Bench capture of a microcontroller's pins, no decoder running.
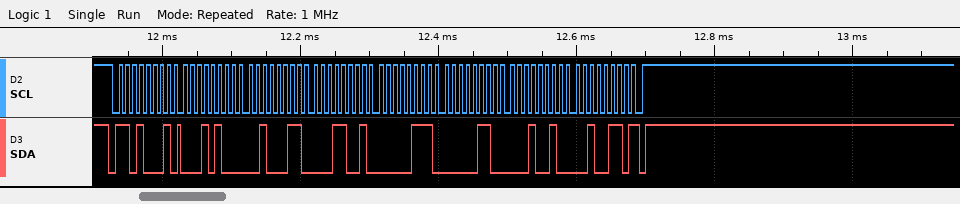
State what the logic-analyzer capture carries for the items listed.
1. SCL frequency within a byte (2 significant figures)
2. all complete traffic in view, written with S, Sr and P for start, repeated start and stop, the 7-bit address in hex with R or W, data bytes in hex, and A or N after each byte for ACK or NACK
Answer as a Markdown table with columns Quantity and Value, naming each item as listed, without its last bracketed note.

| Quantity | Value |
|---|---|
| SCL frequency within a byte | 100 kHz |
| all complete traffic in view, written with S, Sr and P for start, repeated start and stop, the 7-bit address in hex with R or W, data bytes in hex, and A or N after each byte for ACK or NACK | S 68R A 14 A 23 A 19 A 07 A 06 A 12 A 26 N P |
